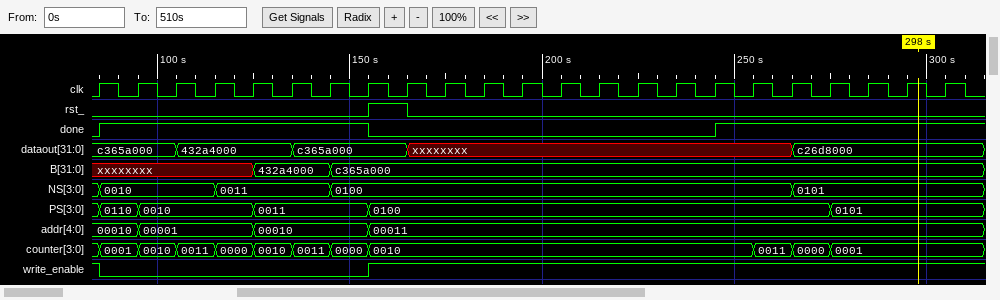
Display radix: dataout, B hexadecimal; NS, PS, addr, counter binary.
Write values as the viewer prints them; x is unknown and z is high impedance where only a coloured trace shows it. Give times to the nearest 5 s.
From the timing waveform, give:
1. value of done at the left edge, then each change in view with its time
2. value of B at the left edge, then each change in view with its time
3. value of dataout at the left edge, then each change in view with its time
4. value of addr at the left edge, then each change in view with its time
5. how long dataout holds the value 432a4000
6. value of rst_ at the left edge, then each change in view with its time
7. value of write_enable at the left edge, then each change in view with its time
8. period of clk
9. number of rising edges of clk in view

0, 1 at 85 s, 0 at 155 s, 1 at 245 s
xxxxxxxx, 432a4000 at 125 s, c365a000 at 145 s
c365a000, 432a4000 at 105 s, c365a000 at 135 s, xxxxxxxx at 165 s, c26d8000 at 265 s
00010, 00001 at 95 s, 00010 at 125 s, 00011 at 155 s
30 s
0, 1 at 155 s, 0 at 165 s
1, 0 at 85 s, 1 at 155 s
10 s
23
